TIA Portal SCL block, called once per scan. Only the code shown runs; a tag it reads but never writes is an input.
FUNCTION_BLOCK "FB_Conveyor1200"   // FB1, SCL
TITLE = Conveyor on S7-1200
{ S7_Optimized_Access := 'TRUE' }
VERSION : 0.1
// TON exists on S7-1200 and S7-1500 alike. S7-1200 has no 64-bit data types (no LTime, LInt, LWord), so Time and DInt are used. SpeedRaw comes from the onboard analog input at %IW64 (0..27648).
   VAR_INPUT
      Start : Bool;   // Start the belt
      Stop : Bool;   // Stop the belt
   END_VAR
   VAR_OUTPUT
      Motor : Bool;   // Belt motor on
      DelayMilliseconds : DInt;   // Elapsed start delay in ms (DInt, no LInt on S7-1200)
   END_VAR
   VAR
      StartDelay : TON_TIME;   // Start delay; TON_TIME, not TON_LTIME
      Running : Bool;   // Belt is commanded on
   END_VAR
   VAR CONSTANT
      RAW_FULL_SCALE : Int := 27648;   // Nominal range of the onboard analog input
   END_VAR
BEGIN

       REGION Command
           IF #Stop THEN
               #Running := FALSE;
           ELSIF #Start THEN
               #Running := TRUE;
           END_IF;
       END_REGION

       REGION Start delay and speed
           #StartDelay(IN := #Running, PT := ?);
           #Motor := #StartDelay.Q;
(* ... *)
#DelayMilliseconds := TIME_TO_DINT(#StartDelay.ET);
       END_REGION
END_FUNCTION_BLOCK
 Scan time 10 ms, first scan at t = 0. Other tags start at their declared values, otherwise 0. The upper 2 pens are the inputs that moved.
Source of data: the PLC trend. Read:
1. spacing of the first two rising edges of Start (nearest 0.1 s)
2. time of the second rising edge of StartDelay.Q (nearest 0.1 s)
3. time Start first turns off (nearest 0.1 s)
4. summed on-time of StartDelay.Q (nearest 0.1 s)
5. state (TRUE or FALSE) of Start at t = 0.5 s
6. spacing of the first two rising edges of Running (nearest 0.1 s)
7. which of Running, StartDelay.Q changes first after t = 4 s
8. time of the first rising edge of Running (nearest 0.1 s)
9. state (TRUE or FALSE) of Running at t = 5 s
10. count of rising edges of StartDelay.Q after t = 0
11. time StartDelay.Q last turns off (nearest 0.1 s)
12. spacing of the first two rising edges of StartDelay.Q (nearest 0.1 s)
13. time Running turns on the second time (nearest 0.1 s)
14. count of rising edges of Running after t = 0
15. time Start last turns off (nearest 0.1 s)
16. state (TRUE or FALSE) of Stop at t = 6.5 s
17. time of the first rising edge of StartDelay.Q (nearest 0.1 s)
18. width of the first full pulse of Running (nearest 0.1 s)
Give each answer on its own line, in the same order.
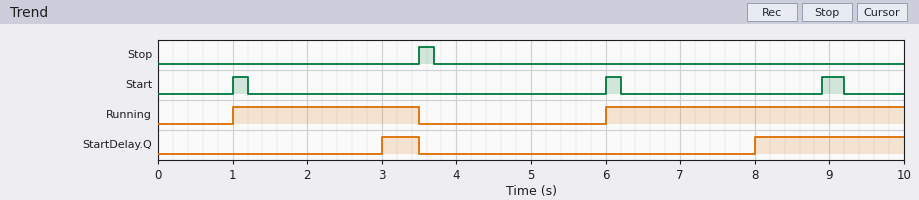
5.0 s
8.0 s
1.2 s
2.5 s
FALSE
5.0 s
Running
1.0 s
FALSE
2
3.5 s
5.0 s
6.0 s
2
9.2 s
FALSE
3.0 s
2.5 s
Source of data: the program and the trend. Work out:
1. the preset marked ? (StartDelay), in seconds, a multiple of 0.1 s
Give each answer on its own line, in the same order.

2.0 s
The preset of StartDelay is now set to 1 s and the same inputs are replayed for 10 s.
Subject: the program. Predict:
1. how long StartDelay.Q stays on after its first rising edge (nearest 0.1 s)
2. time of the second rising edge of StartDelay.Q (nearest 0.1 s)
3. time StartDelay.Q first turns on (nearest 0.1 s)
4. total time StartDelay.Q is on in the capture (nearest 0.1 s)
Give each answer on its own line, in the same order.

1.5 s
7.0 s
2.0 s
4.5 s
